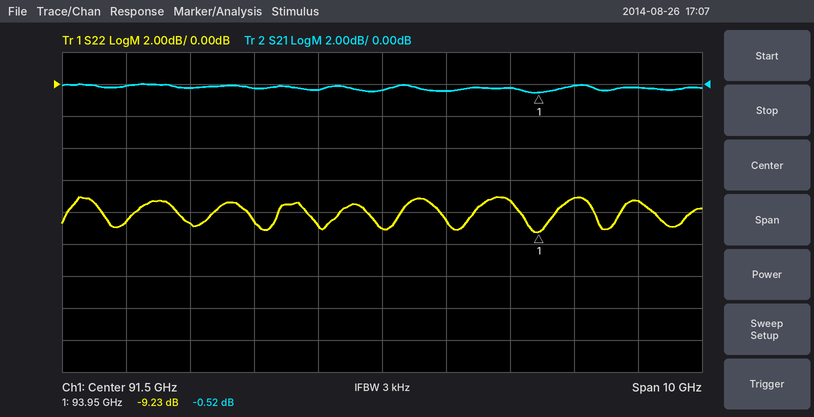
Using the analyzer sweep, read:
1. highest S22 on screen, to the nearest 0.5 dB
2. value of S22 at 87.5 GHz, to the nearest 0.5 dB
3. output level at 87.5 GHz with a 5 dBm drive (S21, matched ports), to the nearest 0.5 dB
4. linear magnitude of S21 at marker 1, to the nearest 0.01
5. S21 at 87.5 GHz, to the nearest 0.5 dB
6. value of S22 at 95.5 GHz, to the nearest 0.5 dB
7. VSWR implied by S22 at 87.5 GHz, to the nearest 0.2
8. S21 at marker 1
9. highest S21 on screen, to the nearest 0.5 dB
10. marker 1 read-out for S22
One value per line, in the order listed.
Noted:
-7.0 dB
-8.5 dB
5.0 dBm
0.94
0.0 dB
-7.5 dB
2.2
-0.52 dB
0.0 dB
-9.23 dB
